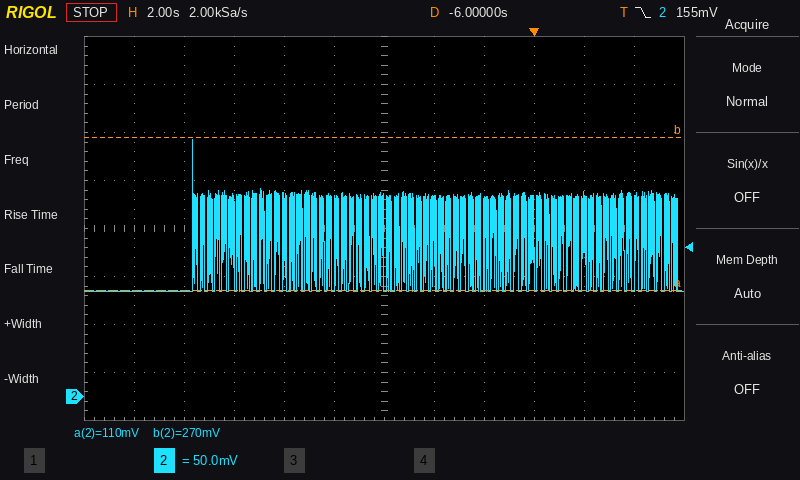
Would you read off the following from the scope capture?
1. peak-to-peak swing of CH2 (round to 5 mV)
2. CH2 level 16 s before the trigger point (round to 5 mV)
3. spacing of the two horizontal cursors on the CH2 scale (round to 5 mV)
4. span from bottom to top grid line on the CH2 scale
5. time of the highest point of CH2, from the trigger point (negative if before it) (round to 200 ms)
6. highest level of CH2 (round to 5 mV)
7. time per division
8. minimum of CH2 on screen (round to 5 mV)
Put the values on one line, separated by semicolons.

160 mV; 110 mV; 160 mV; 400 mV; -13.6 s; 270 mV; 2 s; 110 mV
